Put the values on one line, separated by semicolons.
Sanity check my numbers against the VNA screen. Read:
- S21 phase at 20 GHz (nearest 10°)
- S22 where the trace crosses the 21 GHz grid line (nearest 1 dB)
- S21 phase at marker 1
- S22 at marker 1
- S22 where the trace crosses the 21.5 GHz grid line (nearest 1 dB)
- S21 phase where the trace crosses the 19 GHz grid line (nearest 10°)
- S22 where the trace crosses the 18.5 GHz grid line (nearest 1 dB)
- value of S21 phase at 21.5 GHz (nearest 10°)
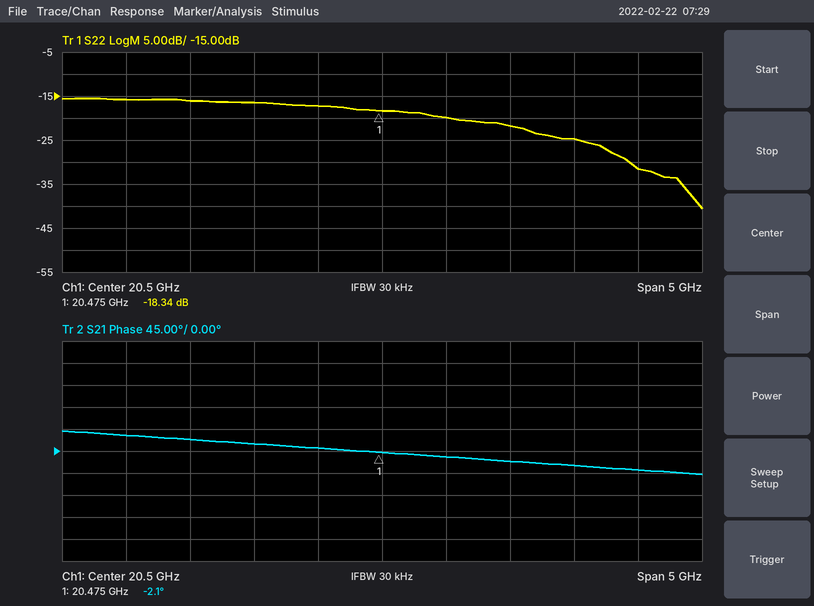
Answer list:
10°; -20 dB; -2.1°; -18.34 dB; -22 dB; 20°; -16 dB; -20°
